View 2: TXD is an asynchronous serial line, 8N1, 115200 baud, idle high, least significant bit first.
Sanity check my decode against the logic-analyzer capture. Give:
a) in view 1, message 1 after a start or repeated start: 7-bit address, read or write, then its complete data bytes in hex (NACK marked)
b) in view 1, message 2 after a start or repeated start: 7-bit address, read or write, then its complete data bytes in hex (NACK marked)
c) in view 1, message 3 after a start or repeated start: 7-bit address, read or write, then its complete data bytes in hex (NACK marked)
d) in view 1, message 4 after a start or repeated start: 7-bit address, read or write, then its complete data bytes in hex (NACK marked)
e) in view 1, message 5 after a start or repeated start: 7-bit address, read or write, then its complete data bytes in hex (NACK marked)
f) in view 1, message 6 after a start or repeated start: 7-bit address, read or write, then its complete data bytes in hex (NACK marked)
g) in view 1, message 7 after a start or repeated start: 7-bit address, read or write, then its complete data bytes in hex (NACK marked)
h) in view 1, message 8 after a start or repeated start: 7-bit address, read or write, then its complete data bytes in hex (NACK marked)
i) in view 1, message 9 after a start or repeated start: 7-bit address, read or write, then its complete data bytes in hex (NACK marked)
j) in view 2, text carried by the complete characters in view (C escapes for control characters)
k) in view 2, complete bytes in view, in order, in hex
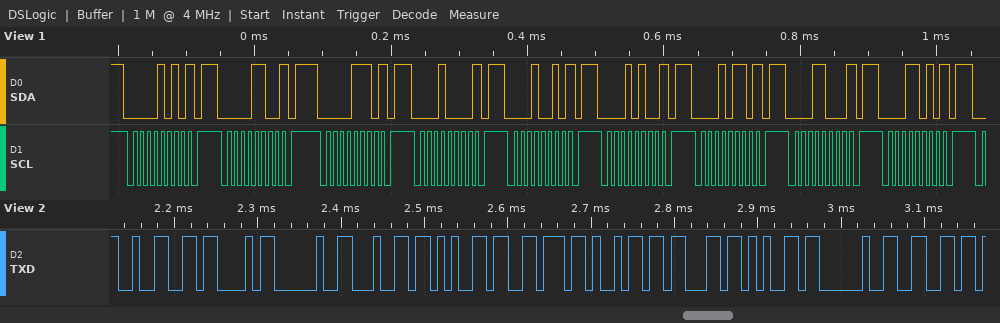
0x05 write NACK
0x06 write NACK
0x07 write NACK
0x08 write NACK
0x09 write NACK
0x0A write NACK
0x0B write NACK
0x0C write NACK
0x0D write NACK
"2C device f"
32 43 20 64 65 76 69 63 65 20 66
